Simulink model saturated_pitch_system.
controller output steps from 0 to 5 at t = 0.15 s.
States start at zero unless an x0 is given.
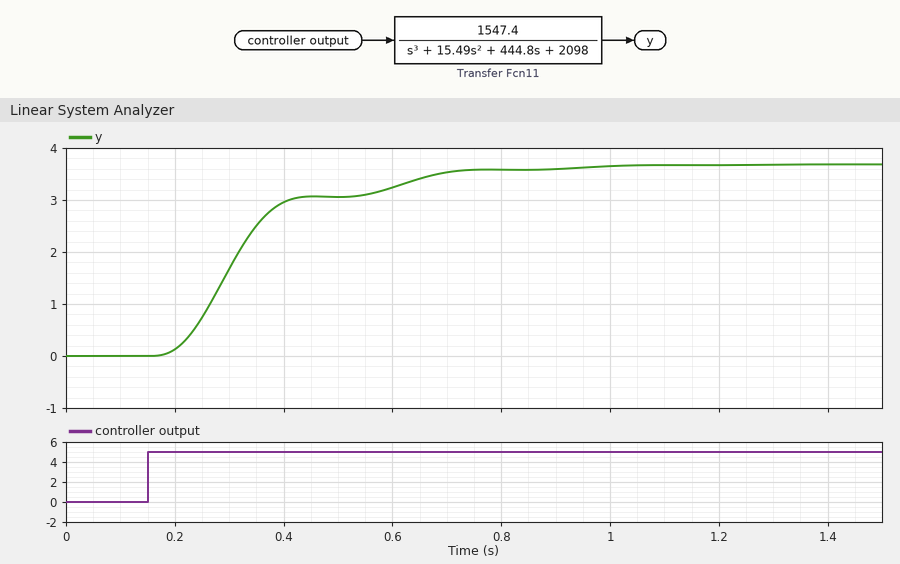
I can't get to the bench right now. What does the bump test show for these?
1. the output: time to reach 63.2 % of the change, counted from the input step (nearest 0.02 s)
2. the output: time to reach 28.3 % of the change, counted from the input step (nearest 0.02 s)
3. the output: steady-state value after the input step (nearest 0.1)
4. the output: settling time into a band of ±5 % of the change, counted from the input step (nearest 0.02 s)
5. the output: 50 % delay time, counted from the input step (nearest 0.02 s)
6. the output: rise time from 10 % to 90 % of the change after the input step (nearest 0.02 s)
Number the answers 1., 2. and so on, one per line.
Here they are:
1. 0.18 s
2. 0.12 s
3. 3.7
4. 0.54 s
5. 0.16 s
6. 0.40 s
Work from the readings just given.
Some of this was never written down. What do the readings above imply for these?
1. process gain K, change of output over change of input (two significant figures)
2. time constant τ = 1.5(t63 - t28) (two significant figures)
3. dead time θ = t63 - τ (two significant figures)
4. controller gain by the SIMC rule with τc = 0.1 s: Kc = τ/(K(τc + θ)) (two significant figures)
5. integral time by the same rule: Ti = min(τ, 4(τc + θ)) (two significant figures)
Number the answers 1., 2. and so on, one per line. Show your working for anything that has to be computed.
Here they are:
1. (3.7 - 0) / 5 = 0.74
2. 1.5 × (0.18 - 0.12) = 0.090 s
3. 0.18 - 0.09 = 0.090 s
4. 0.09 / (0.74 × (0.1 + 0.09)) = 0.64
5. min(0.09, 4 × (0.1 + 0.09)) = 0.090 s
